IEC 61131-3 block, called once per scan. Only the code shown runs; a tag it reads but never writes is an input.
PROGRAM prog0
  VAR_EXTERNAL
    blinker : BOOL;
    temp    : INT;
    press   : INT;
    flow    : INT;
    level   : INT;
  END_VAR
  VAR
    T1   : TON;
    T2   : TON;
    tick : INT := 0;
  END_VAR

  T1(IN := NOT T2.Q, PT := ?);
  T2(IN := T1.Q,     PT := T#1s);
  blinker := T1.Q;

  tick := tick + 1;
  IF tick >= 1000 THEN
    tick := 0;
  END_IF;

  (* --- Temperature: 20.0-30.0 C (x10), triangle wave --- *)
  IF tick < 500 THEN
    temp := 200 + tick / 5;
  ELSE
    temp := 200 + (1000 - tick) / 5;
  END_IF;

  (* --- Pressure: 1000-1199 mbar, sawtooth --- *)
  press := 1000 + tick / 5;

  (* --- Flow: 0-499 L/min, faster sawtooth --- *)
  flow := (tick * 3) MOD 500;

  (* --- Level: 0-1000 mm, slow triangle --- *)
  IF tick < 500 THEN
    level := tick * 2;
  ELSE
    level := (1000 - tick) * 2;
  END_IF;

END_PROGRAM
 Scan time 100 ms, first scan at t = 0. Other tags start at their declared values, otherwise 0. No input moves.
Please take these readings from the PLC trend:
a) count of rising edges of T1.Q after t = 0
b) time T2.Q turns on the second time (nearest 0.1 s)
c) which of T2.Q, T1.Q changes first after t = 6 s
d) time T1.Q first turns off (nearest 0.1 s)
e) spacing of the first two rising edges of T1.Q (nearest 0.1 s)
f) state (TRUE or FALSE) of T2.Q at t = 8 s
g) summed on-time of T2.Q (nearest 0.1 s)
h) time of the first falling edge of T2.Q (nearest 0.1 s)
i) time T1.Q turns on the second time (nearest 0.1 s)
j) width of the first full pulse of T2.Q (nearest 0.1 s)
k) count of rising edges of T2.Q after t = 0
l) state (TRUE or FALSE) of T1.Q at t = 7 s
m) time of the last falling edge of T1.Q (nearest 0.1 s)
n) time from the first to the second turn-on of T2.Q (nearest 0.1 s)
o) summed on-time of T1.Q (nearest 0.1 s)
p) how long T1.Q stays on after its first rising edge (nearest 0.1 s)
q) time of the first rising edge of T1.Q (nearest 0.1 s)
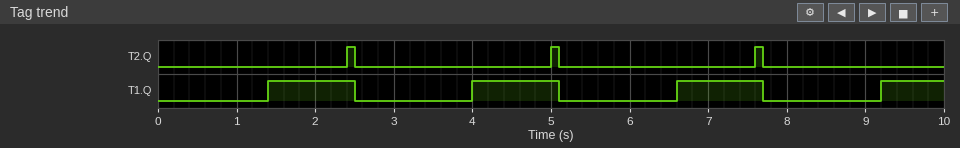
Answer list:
4
5.0 s
T1.Q
2.5 s
2.6 s
FALSE
0.3 s
2.5 s
4.0 s
0.1 s
3
TRUE
7.7 s
2.6 s
4.1 s
1.1 s
1.4 s
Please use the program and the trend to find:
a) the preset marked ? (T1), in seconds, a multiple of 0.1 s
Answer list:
1.4 s
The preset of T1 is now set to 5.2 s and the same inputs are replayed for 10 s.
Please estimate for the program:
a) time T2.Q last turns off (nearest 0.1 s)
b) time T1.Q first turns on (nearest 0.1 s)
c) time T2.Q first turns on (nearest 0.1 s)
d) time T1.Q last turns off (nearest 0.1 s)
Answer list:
6.3 s
5.2 s
6.2 s
6.3 s
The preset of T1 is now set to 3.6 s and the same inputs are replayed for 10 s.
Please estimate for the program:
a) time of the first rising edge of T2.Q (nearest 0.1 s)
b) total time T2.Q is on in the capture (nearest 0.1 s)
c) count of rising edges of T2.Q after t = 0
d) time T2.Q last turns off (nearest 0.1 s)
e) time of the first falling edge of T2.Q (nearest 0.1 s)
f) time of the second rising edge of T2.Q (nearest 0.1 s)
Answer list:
4.6 s
0.2 s
2
9.5 s
4.7 s
9.4 s
